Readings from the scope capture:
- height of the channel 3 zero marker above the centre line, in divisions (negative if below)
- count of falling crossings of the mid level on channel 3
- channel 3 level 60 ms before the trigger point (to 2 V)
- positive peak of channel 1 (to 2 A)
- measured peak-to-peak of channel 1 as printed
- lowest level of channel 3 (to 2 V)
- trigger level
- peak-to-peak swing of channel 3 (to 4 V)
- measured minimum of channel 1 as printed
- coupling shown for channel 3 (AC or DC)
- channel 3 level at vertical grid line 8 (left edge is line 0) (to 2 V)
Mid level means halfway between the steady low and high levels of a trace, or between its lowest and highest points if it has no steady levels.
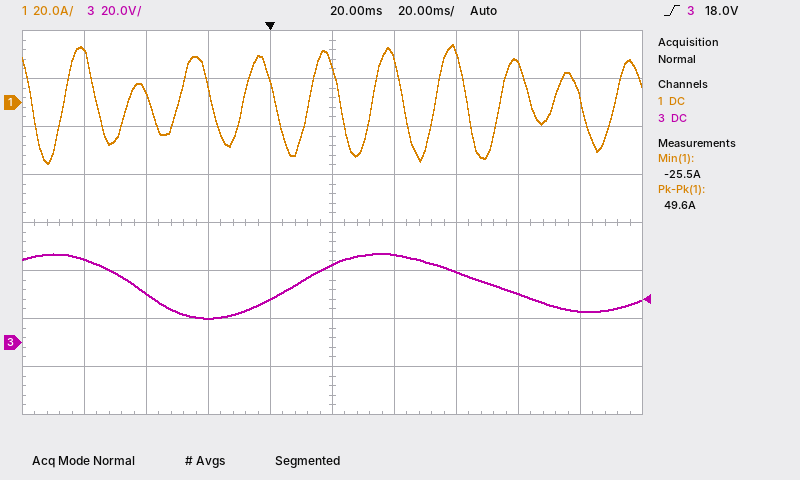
-2.5 div
2
34 V
24 A
49.6 A
10 V
18.0 V
28 V
-25.5 A
DC
20 V
